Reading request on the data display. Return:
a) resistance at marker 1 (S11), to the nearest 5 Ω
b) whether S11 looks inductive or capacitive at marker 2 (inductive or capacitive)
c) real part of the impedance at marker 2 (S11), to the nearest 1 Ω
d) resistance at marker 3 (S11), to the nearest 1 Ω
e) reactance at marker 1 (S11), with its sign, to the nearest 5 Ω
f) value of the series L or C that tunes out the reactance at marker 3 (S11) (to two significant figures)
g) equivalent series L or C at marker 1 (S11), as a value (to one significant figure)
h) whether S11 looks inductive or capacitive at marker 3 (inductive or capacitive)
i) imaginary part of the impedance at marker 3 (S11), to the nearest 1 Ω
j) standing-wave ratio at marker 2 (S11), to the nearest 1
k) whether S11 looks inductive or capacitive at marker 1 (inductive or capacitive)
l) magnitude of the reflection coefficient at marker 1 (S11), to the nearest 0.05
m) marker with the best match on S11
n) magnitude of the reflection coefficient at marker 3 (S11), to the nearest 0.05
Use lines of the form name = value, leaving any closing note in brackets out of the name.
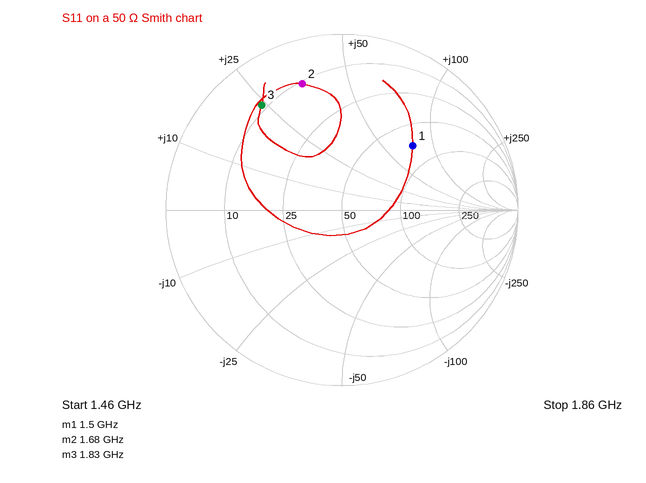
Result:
resistance at marker 1 (S11), to the nearest 5 Ω = 70 Ω
whether S11 looks inductive or capacitive at marker 2 = inductive
real part of the impedance at marker 2 (S11), to the nearest 1 Ω = 11 Ω
resistance at marker 3 (S11), to the nearest 1 Ω = 9 Ω
reactance at marker 1 (S11), with its sign, to the nearest 5 Ω = +75 Ω
value of the series L or C that tunes out the reactance at marker 3 (S11) = 3.6 pF
equivalent series L or C at marker 1 (S11), as a value = 8 nH
whether S11 looks inductive or capacitive at marker 3 = inductive
imaginary part of the impedance at marker 3 (S11), to the nearest 1 Ω = +24 Ω
standing-wave ratio at marker 2 (S11), to the nearest 1 = 7
whether S11 looks inductive or capacitive at marker 1 = inductive
magnitude of the reflection coefficient at marker 1 (S11), to the nearest 0.05 = 0.55
marker with the best match on S11 = marker 1
magnitude of the reflection coefficient at marker 3 (S11), to the nearest 0.05 = 0.75
